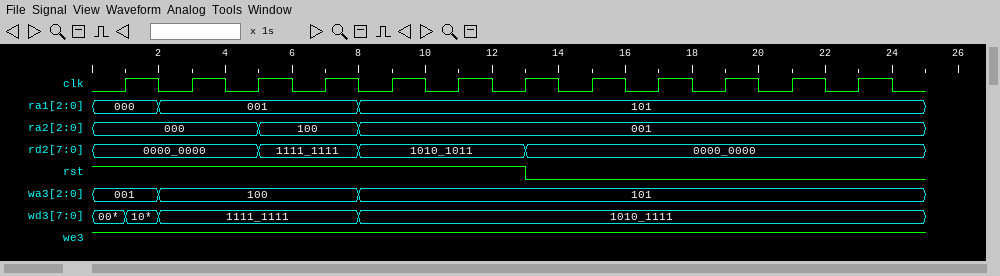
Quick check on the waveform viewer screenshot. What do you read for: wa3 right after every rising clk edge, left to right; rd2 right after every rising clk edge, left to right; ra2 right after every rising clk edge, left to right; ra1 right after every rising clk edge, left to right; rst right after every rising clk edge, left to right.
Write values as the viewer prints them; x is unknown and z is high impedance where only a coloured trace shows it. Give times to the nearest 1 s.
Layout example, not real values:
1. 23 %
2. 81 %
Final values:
1. 001, 100, 100, 100, 101, 101, 101, 101, 101, 101, 101, 101
2. 0000_0000, 0000_0000, 1111_1111, 1111_1111, 1010_1011, 1010_1011, 0000_0000, 0000_0000, 0000_0000, 0000_0000, 0000_0000, 0000_0000
3. 000, 000, 100, 100, 001, 001, 001, 001, 001, 001, 001, 001
4. 000, 001, 001, 001, 101, 101, 101, 101, 101, 101, 101, 101
5. 1 1 1 1 1 1 0 0 0 0 0 0
